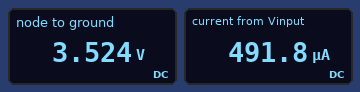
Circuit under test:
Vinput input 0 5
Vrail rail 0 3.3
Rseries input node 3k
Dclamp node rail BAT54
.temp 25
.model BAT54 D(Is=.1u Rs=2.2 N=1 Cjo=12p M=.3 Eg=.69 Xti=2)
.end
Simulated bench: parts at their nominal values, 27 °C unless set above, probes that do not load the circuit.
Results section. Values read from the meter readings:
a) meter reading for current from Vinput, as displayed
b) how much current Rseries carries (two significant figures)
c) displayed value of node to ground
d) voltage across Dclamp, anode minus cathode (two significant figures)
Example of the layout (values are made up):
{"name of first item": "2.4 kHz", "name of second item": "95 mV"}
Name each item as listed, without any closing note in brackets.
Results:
{"meter reading for current from Vinput, as displayed": "491.8 µA", "how much current Rseries carries": "490 µA", "displayed value of node to ground": "3.524 V", "voltage across Dclamp, anode minus cathode": "220 mV"}
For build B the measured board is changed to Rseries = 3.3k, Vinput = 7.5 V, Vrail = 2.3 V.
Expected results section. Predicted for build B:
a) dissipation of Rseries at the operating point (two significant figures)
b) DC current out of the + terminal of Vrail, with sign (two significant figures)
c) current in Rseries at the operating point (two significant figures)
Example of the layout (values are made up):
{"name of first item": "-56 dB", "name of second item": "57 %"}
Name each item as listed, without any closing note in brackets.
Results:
{"dissipation of Rseries at the operating point": "7.4 mW", "DC current out of the + terminal of Vrail, with sign": "-1.5 mA", "current in Rseries at the operating point": "1.5 mA"}
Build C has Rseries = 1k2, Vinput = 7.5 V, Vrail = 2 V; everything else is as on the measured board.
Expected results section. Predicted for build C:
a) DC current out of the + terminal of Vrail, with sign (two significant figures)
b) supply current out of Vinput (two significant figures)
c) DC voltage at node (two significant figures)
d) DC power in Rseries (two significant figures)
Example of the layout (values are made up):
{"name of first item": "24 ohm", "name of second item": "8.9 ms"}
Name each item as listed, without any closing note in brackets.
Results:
{"DC current out of the + terminal of Vrail, with sign": "-4.3 mA", "supply current out of Vinput": "4.3 mA", "DC voltage at node": "2.3 V", "DC power in Rseries": "23 mW"}
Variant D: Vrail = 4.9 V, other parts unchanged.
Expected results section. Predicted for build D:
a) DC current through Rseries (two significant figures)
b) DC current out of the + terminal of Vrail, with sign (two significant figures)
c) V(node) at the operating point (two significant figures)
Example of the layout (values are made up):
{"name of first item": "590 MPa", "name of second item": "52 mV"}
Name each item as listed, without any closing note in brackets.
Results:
{"DC current through Rseries": "2.8 µA", "DC current out of the + terminal of Vrail, with sign": "-2.8 µA", "V(node) at the operating point": "5.0 V"}
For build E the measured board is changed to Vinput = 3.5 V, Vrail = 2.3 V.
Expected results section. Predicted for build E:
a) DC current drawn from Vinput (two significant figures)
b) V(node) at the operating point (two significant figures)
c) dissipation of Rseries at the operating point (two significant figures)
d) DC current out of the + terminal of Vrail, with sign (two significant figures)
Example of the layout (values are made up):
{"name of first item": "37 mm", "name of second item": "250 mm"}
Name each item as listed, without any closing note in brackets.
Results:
{"DC current drawn from Vinput": "330 µA", "V(node) at the operating point": "2.5 V", "dissipation of Rseries at the operating point": "320 µW", "DC current out of the + terminal of Vrail, with sign": "-330 µA"}
